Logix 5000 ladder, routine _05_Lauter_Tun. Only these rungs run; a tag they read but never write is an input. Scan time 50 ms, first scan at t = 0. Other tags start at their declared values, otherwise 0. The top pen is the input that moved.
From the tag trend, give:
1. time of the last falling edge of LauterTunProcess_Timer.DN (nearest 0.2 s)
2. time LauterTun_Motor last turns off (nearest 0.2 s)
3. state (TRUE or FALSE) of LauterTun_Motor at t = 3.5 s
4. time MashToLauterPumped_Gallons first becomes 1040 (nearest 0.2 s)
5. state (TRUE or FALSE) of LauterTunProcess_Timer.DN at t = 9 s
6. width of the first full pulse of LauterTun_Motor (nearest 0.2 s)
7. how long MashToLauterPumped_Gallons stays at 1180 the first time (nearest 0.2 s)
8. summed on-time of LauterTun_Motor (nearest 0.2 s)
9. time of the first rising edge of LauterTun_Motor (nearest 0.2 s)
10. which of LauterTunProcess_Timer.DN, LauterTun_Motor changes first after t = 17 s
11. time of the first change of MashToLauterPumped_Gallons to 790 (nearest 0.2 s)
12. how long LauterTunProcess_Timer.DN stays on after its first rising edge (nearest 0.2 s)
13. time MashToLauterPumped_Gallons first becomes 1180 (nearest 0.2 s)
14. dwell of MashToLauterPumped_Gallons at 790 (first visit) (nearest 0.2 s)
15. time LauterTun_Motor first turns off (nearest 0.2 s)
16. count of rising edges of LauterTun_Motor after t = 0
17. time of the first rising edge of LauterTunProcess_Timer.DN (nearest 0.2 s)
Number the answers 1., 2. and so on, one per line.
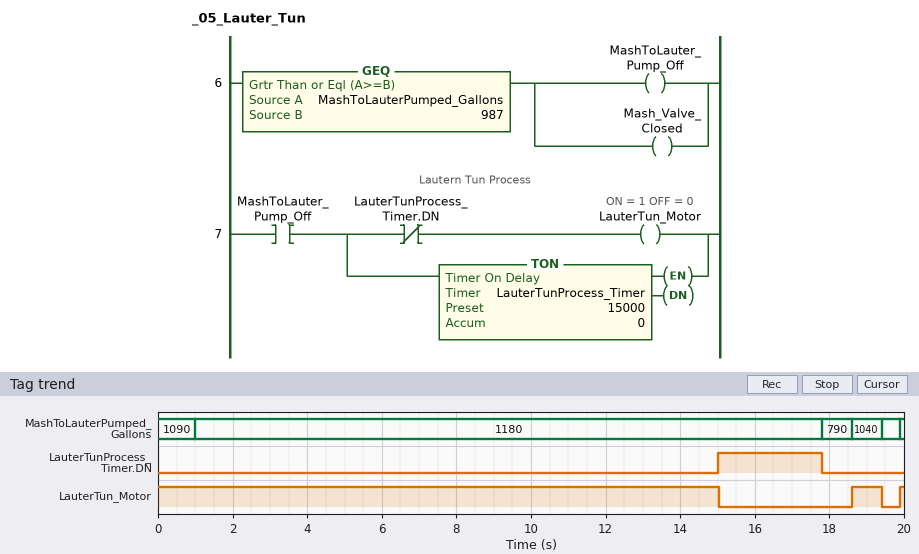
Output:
1. 17.8 s
2. 19.4 s
3. TRUE
4. 18.6 s
5. FALSE
6. 0.8 s
7. 16.8 s
8. 16.0 s
9. 18.6 s
10. LauterTunProcess_Timer.DN
11. 17.8 s
12. 2.8 s
13. 1.0 s
14. 0.8 s
15. 15.0 s
16. 2
17. 15.0 s
